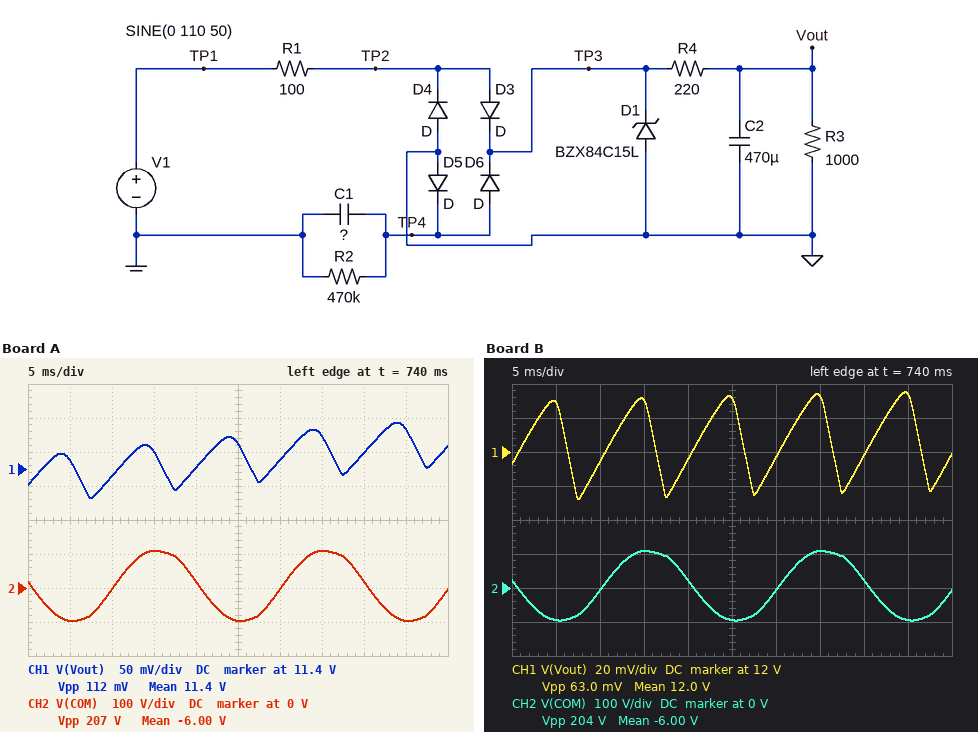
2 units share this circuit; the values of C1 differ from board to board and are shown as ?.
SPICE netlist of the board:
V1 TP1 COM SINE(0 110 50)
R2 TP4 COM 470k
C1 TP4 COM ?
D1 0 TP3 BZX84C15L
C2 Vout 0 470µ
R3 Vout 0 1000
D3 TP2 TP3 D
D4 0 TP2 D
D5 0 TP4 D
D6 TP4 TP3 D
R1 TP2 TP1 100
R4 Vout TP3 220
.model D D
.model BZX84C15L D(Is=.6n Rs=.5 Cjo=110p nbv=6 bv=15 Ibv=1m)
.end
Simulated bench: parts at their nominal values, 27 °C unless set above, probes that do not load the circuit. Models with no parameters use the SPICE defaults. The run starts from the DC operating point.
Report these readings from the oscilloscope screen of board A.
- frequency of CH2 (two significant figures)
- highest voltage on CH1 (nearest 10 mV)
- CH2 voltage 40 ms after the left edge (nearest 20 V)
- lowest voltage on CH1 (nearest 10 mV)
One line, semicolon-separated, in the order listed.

50 Hz; 11.47 V; 20 V; 11.36 V
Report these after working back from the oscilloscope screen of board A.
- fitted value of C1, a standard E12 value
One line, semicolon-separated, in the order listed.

820 nF
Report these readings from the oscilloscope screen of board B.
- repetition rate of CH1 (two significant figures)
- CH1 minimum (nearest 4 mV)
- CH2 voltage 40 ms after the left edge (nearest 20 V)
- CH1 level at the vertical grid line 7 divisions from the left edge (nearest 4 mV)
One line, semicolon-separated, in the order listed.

100 Hz; 11.972 V; 20 V; 12.032 V
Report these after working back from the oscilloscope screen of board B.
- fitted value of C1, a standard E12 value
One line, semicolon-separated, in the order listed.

1.8 µF
